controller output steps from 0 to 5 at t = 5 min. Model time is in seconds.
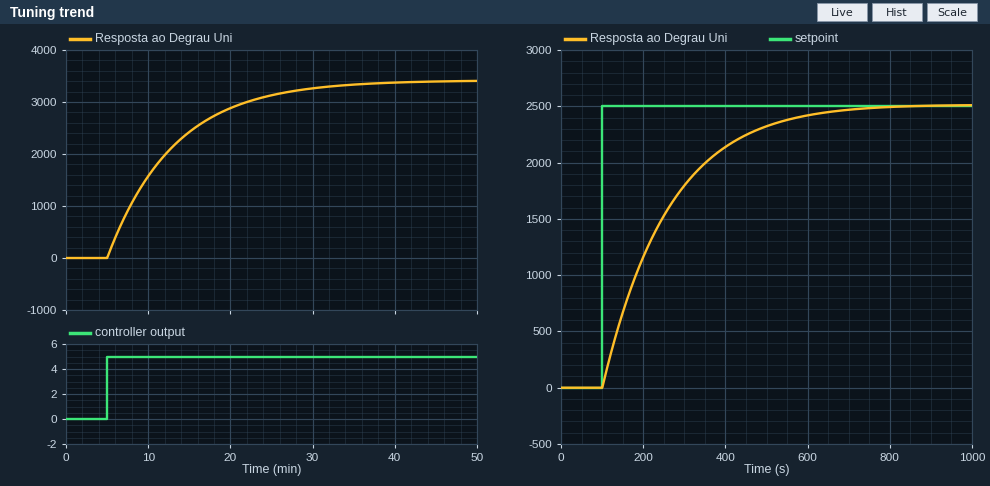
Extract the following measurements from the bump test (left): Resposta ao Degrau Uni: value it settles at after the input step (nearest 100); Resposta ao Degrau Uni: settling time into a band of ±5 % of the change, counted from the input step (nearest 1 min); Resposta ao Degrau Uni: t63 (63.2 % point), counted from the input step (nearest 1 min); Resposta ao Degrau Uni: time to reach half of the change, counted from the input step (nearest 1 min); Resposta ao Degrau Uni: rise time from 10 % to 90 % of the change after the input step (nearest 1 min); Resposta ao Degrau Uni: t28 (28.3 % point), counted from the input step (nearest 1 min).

3400
24 min
8 min
6 min
18 min
3 min
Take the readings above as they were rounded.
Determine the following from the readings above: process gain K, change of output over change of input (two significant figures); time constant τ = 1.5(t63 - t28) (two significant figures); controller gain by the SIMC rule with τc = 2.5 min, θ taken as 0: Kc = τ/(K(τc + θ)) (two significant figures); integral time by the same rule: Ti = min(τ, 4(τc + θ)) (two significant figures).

680
7.5 min
0.0044
7.5 min
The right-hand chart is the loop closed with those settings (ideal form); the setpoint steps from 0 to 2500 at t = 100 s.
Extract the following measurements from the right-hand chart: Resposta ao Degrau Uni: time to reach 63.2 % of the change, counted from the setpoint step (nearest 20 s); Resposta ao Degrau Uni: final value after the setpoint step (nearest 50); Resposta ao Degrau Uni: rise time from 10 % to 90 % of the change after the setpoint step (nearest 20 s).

160 s
2500
340 s
